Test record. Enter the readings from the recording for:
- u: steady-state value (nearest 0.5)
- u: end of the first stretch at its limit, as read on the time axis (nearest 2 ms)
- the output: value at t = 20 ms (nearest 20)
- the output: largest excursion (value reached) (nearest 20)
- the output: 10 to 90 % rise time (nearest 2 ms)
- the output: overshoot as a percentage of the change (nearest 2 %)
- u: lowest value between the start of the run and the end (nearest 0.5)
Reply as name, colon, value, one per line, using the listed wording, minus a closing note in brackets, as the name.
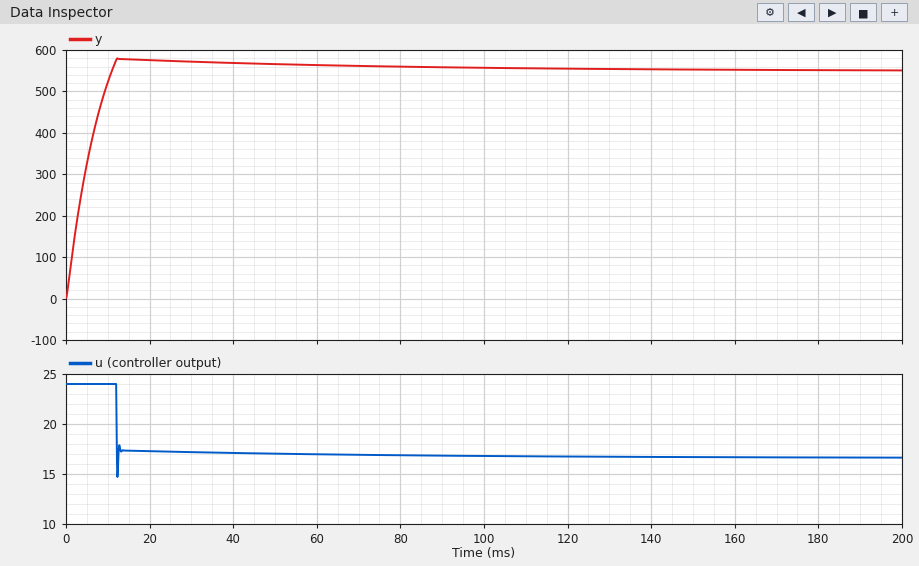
u: steady-state value: 16.5
u: end of the first stretch at its limit, as read on the time axis: 12 ms
the output: value at t = 20 ms: 580
the output: largest excursion (value reached): 580
the output: 10 to 90 % rise time: 8 ms
the output: overshoot as a percentage of the change: 6 %
u: lowest value between the start of the run and the end: 14.5
